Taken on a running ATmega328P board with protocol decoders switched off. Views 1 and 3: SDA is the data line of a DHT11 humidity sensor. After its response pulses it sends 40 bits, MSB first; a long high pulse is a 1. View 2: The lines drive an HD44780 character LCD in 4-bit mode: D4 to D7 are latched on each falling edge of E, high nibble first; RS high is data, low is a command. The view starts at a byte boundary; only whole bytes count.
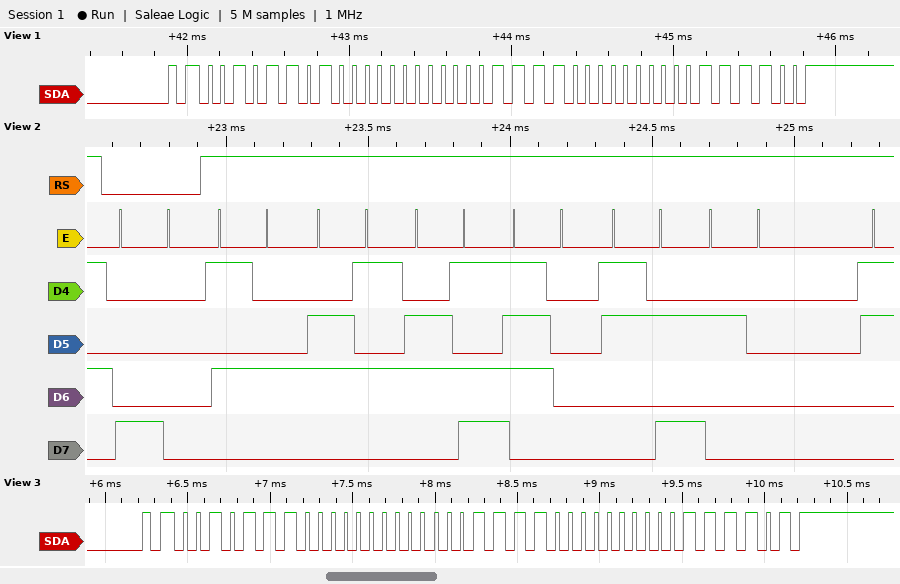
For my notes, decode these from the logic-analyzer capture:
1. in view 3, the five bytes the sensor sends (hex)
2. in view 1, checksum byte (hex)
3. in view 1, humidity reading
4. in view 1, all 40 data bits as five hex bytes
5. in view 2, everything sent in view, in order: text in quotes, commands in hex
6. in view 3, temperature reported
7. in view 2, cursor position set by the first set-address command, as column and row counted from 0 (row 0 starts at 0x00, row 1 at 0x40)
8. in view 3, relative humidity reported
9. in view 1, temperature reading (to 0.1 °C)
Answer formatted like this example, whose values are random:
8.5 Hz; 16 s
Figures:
2E 00 0F 00 3D; 0x3C; 45 %; 2D 00 0F 00 3C; 0x80 "Temp: "; 15.0 °C; column 0, row 0; 46 %; 15.0 °C
